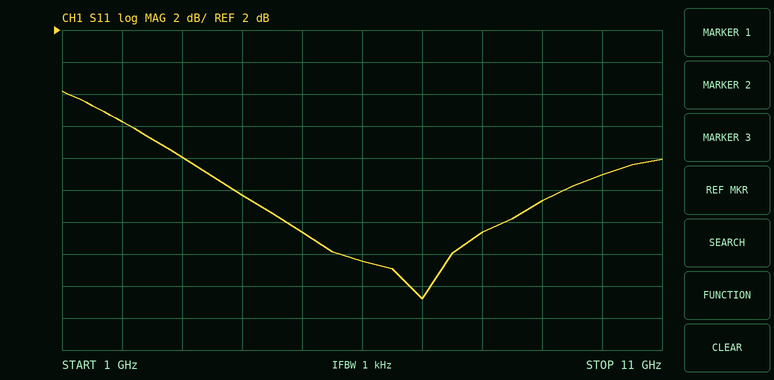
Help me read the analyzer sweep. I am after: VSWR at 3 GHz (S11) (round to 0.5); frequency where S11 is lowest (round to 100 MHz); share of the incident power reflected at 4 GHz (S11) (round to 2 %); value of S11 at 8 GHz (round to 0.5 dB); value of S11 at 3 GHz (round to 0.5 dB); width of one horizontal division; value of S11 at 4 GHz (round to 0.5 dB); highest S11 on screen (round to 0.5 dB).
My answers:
3.0
7.0 GHz
14 %
-10.5 dB
-6.0 dB
1 GHz
-8.5 dB
-2.0 dB
